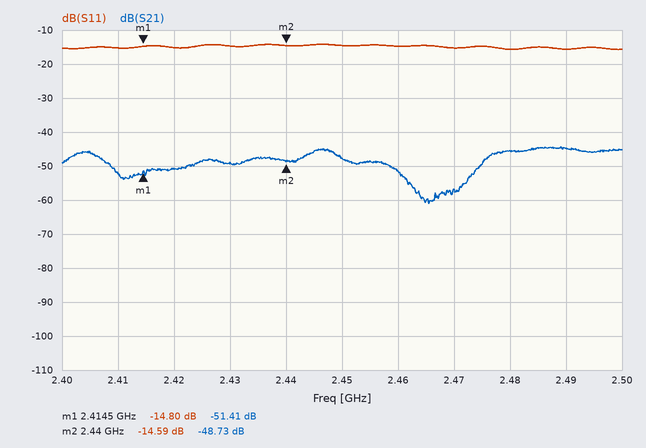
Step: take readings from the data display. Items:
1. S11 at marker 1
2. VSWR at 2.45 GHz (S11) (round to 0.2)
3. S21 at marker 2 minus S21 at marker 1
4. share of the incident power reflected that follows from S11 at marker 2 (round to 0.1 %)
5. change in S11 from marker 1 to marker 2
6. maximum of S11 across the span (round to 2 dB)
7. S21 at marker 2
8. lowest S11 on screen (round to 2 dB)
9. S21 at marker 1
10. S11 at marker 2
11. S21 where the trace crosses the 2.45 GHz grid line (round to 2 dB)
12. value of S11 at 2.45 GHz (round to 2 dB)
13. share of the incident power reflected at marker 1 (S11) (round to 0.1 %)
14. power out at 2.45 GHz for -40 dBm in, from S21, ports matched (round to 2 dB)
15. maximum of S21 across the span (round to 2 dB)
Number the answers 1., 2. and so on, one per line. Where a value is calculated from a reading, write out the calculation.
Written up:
1. -14.80 dB
2. |Γ| = 10^(-14/20) = 0.1995; VSWR = (1 + 0.1995)/(1 − 0.1995) ≈ 1.50, so 1.4 to the nearest 0.2
3. -48.73 − (-51.41) = 2.68 dB
4. 10^(-14.59/10) ≈ 3.5 %
5. -14.59 − (-14.8) = 0.21 dB
6. -14 dB
7. -48.73 dB
8. -16 dB
9. -51.41 dB
10. -14.59 dB
11. -48 dB
12. -14 dB
13. 10^(-14.8/10) ≈ 3.3 %
14. -40 dBm + (-48 dB) = -88 dBm
15. -44 dB
